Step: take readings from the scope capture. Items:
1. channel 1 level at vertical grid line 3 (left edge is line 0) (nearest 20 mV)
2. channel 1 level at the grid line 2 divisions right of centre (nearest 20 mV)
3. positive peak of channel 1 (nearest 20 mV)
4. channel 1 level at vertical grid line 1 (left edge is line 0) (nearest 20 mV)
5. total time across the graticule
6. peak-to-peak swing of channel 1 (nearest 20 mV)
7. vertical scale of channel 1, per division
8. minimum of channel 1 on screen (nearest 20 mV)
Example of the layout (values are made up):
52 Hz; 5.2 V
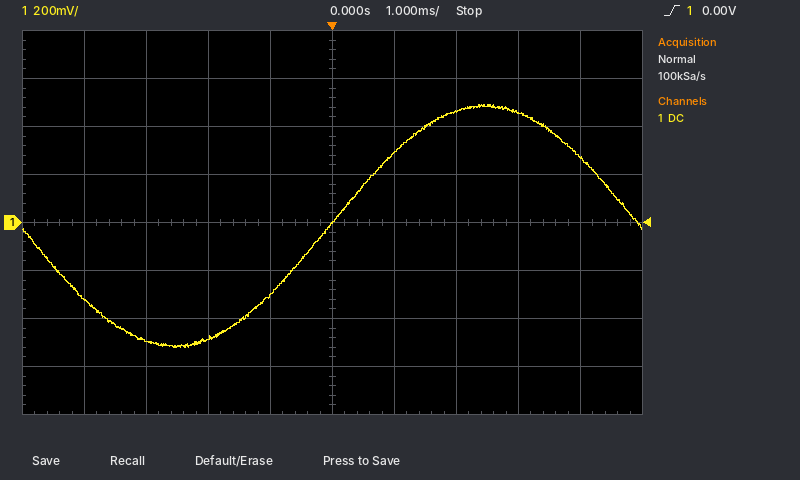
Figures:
-480 mV; 460 mV; 500 mV; -320 mV; 10 ms; 1.02 V; 200 mV; -520 mV
